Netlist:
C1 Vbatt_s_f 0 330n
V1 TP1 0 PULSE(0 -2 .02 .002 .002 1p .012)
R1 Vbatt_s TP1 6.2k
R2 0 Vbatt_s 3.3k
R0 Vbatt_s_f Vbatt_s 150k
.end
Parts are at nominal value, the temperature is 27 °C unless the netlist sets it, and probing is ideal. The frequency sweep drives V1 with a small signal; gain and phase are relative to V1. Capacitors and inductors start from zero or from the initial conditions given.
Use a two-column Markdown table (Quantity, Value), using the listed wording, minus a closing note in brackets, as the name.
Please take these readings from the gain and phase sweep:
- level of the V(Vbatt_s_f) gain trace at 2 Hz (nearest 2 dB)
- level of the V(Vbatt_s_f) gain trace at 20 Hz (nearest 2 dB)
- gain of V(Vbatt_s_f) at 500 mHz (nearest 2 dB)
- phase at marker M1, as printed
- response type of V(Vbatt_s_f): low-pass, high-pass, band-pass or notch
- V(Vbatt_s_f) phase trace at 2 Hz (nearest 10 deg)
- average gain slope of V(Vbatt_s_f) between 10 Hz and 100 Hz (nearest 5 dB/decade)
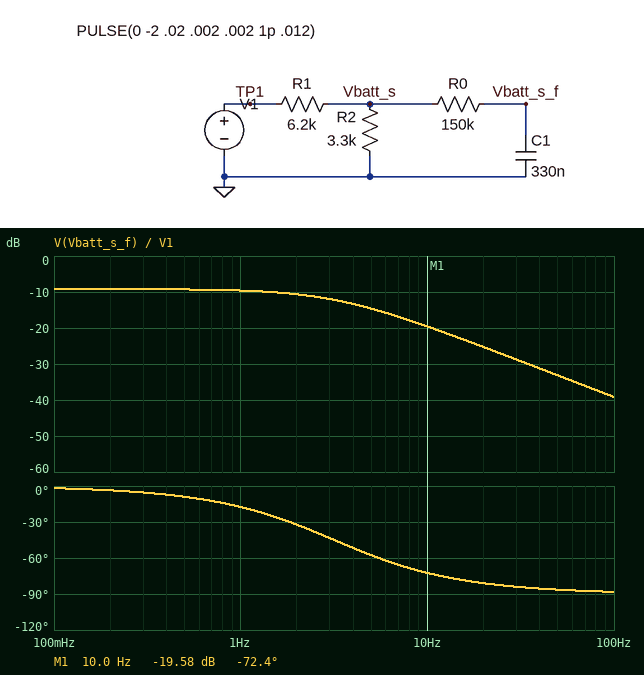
| Quantity | Value |
|---|---|
| level of the V(Vbatt_s_f) gain trace at 2 Hz | -10 dB |
| level of the V(Vbatt_s_f) gain trace at 20 Hz | -26 dB |
| gain of V(Vbatt_s_f) at 500 mHz | -10 dB |
| phase at marker M1, as printed | -72.4 deg |
| response type of V(Vbatt_s_f): low-pass, high-pass, band-pass or notch | low-pass |
| V(Vbatt_s_f) phase trace at 2 Hz | -30 deg |
| average gain slope of V(Vbatt_s_f) between 10 Hz and 100 Hz | -20 dB/decade |
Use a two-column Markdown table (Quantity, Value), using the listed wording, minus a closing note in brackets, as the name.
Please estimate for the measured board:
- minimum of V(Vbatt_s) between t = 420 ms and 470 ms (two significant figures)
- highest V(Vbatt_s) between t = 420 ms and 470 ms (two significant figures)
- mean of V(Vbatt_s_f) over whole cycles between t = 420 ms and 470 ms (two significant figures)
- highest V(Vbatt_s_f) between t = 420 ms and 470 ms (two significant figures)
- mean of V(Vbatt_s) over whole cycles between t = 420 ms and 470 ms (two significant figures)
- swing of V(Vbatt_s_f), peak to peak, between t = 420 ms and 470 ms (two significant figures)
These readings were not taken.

| Quantity | Value |
|---|---|
| minimum of V(Vbatt_s) between t = 420 ms and 470 ms | -690 mV |
| highest V(Vbatt_s) between t = 420 ms and 470 ms | -1.5 mV |
| mean of V(Vbatt_s_f) over whole cycles between t = 420 ms and 470 ms | -120 mV |
| highest V(Vbatt_s_f) between t = 420 ms and 470 ms | -110 mV |
| mean of V(Vbatt_s) over whole cycles between t = 420 ms and 470 ms | -120 mV |
| swing of V(Vbatt_s_f), peak to peak, between t = 420 ms and 470 ms | 19 mV |
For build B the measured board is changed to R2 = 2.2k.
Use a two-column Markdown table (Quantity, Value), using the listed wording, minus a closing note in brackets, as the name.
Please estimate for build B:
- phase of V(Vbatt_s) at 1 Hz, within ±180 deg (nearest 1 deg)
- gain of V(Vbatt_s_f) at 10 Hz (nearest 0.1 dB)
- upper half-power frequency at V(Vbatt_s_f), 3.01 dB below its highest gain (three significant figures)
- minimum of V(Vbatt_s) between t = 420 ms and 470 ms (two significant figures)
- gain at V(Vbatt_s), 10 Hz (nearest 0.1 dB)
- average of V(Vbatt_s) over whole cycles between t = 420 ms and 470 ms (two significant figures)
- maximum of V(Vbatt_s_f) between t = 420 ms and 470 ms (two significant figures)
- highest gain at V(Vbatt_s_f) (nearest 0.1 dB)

| Quantity | Value |
|---|---|
| phase of V(Vbatt_s) at 1 Hz, within ±180 deg | 0 deg |
| gain of V(Vbatt_s_f) at 10 Hz | -22.0 dB |
| upper half-power frequency at V(Vbatt_s_f), 3.01 dB below its highest gain | 3.18 Hz |
| minimum of V(Vbatt_s) between t = 420 ms and 470 ms | -520 mV |
| gain at V(Vbatt_s), 10 Hz | -11.7 dB |
| average of V(Vbatt_s) over whole cycles between t = 420 ms and 470 ms | -87 mV |
| maximum of V(Vbatt_s_f) between t = 420 ms and 470 ms | -80 mV |
| highest gain at V(Vbatt_s_f) | -11.6 dB |
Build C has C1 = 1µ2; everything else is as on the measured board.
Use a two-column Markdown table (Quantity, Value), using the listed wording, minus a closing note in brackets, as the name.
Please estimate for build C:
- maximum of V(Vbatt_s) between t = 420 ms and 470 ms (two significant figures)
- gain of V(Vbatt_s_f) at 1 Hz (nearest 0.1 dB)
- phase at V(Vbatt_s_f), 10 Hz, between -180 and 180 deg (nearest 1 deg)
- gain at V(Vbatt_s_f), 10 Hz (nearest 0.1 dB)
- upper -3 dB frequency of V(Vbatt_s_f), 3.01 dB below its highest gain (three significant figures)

| Quantity | Value |
|---|---|
| maximum of V(Vbatt_s) between t = 420 ms and 470 ms | -1.4 mV |
| gain of V(Vbatt_s_f) at 1 Hz | -12.8 dB |
| phase at V(Vbatt_s_f), 10 Hz, between -180 and 180 deg | -85 deg |
| gain at V(Vbatt_s_f), 10 Hz | -30.4 dB |
| upper -3 dB frequency of V(Vbatt_s_f), 3.01 dB below its highest gain | 872 mHz |
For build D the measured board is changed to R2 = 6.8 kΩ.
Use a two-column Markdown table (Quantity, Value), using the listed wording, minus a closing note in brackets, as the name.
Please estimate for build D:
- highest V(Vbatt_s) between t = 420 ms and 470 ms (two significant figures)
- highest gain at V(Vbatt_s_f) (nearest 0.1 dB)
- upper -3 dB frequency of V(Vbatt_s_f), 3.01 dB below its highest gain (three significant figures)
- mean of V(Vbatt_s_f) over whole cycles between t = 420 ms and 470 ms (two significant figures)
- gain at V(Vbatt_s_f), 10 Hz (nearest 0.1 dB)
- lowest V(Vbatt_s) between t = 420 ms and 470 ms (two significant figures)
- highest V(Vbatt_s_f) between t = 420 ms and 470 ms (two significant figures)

| Quantity | Value |
|---|---|
| highest V(Vbatt_s) between t = 420 ms and 470 ms | -3.4 mV |
| highest gain at V(Vbatt_s_f) | -5.6 dB |
| upper -3 dB frequency of V(Vbatt_s_f), 3.01 dB below its highest gain | 3.15 Hz |
| mean of V(Vbatt_s_f) over whole cycles between t = 420 ms and 470 ms | -170 mV |
| gain at V(Vbatt_s_f), 10 Hz | -16.1 dB |
| lowest V(Vbatt_s) between t = 420 ms and 470 ms | -1.0 V |
| highest V(Vbatt_s_f) between t = 420 ms and 470 ms | -160 mV |
